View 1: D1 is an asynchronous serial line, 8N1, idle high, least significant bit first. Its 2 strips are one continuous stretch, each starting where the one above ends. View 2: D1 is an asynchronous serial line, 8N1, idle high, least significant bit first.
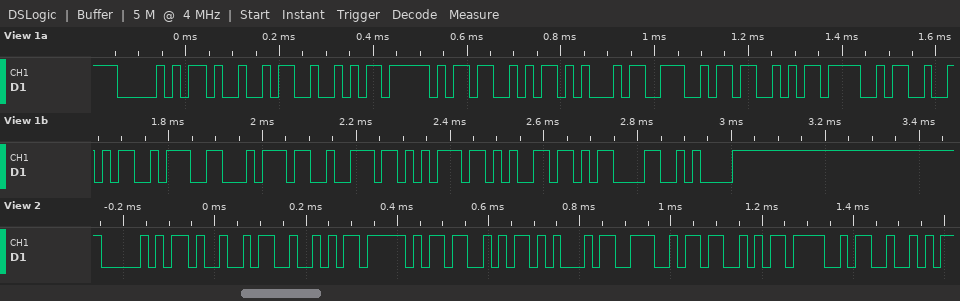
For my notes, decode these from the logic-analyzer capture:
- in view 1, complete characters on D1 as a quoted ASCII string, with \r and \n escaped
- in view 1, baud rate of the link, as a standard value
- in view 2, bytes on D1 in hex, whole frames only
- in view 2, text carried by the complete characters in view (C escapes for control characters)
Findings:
"PIR_SENSOR:true\r\n"
57600 baud
50 49 52 5F 53 45 4E 53 4F 52
"PIR_SENSOR"
